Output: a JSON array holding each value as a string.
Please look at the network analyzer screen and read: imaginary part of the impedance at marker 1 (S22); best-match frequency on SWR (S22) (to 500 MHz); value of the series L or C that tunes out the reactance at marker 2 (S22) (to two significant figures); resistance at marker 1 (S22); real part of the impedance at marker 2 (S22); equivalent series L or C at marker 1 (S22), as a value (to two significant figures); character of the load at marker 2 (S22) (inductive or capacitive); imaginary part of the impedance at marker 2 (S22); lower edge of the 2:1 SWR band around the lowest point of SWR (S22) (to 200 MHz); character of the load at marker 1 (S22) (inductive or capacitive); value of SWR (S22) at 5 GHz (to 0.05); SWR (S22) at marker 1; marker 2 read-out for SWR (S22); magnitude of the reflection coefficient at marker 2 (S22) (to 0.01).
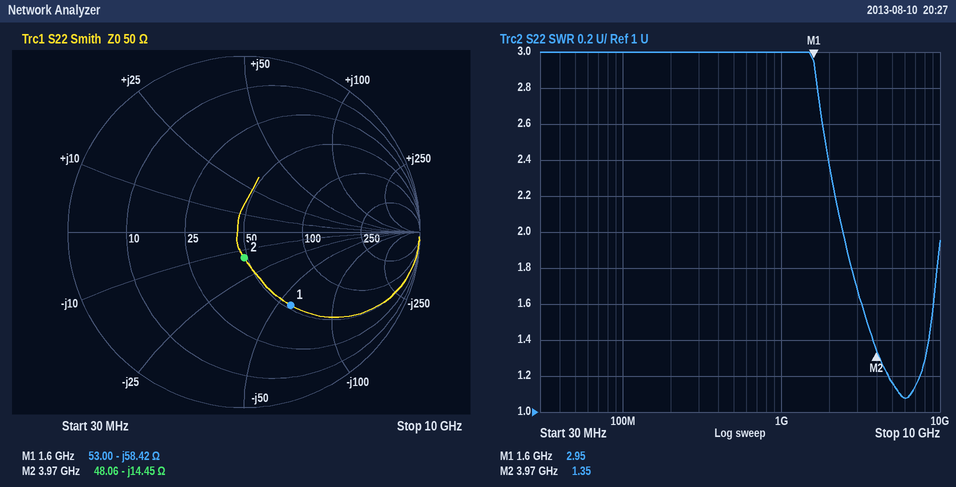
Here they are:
["-58.42 Ω", "6.0 GHz", "580 pH", "53.00 Ω", "48.06 Ω", "1.7 pF", "capacitive", "-14.45 Ω", "2.4 GHz", "capacitive", "1.15", "2.95", "1.35", "0.15"]
